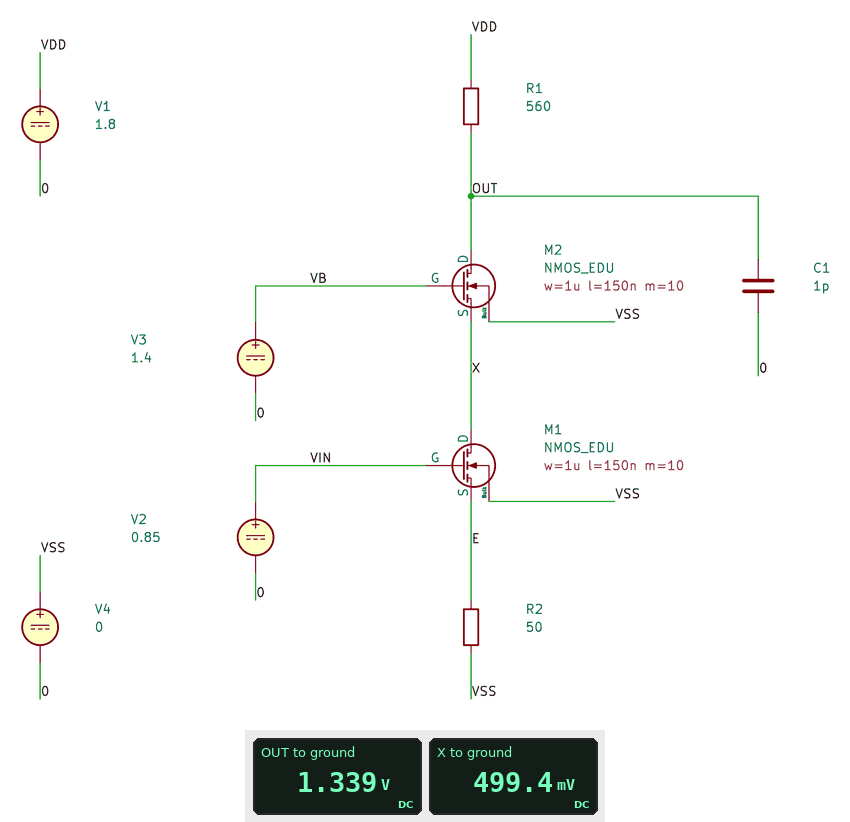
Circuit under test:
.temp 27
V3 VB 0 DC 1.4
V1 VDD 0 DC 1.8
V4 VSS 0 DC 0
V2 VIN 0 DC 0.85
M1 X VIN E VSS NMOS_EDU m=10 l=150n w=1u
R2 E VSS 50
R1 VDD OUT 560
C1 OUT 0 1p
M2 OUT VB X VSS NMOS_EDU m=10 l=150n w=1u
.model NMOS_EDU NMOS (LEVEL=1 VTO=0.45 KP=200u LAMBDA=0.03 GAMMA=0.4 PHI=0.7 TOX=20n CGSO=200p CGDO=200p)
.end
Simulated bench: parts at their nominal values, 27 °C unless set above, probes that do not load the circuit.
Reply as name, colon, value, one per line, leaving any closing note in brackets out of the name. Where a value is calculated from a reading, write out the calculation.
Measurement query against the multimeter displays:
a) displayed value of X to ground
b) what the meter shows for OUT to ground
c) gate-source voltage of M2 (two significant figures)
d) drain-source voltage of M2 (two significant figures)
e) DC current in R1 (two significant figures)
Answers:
displayed value of X to ground: 499.4 mV
what the meter shows for OUT to ground: 1.339 V
gate-source voltage of M2: 1.4 V - 499.4 mV = 900 mV
drain-source voltage of M2: 1.339 V - 499.4 mV = 840 mV
DC current in R1: (1.8 V - 1.339 V) / 560 Ω = 820 µA
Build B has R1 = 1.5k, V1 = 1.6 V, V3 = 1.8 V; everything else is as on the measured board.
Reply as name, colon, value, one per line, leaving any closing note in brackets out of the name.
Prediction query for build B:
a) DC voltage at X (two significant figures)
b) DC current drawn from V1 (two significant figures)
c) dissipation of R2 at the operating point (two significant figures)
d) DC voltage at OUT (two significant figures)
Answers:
DC voltage at X: 330 mV
DC current drawn from V1: 800 µA
dissipation of R2 at the operating point: 32 µW
DC voltage at OUT: 400 mV
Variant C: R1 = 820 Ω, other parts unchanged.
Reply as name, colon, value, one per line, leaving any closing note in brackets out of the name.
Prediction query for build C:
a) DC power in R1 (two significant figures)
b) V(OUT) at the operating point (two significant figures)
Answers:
DC power in R1: 560 µW
V(OUT) at the operating point: 1.1 V
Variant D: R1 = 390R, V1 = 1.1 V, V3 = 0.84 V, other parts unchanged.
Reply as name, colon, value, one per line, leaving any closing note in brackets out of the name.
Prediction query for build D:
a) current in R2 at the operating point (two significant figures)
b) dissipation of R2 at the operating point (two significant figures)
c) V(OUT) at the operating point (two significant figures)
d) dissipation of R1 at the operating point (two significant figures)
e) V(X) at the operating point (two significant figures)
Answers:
current in R2 at the operating point: 420 µA
dissipation of R2 at the operating point: 8.7 µW
V(OUT) at the operating point: 940 mV
dissipation of R1 at the operating point: 68 µW
V(X) at the operating point: 120 mV
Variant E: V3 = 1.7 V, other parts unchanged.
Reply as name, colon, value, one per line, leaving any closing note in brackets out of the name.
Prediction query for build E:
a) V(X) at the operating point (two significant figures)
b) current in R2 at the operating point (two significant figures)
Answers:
V(X) at the operating point: 750 mV
current in R2 at the operating point: 830 µA
